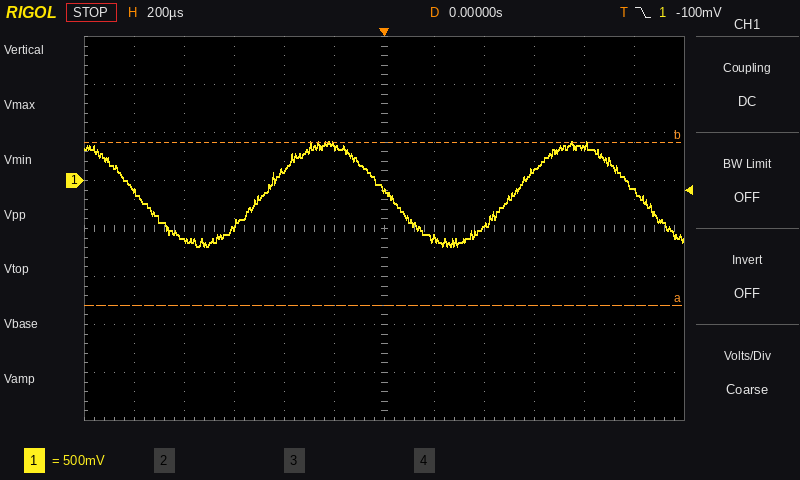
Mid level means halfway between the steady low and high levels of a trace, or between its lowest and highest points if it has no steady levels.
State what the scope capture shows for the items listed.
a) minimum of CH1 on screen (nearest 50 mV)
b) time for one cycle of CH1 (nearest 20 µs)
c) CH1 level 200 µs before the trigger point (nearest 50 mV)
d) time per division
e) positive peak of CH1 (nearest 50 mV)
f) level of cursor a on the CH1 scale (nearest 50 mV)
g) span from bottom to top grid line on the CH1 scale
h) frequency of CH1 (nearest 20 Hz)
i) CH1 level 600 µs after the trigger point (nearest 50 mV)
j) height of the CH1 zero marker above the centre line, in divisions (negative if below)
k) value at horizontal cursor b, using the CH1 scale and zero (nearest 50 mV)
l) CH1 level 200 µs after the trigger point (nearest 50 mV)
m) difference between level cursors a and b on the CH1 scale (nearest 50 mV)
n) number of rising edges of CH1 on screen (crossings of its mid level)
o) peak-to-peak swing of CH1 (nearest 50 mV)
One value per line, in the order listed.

-700 mV
1.00 ms
350 mV
200 µs
400 mV
-1.30 V
4 V
1.00 kHz
100 mV
+1.0 div
400 mV
-600 mV
1.70 V
2
1.10 V
